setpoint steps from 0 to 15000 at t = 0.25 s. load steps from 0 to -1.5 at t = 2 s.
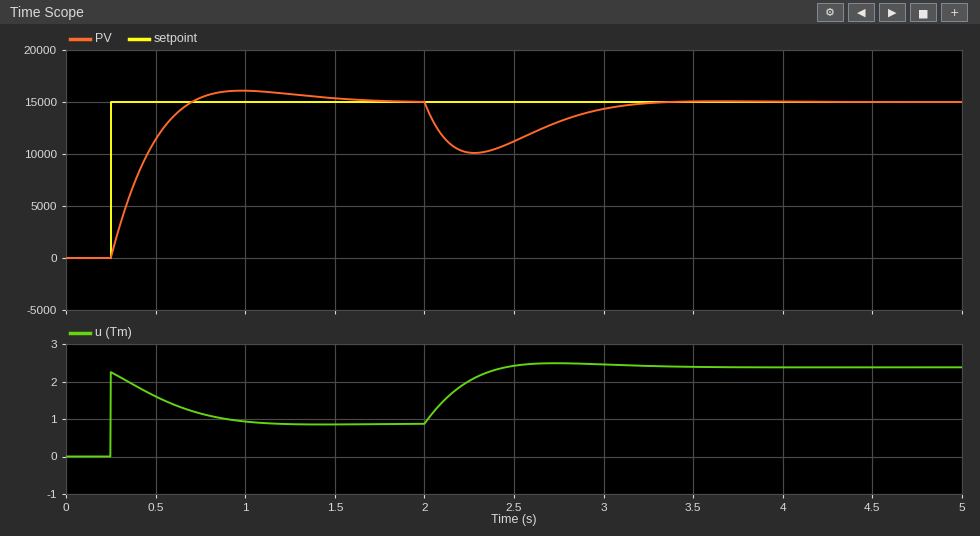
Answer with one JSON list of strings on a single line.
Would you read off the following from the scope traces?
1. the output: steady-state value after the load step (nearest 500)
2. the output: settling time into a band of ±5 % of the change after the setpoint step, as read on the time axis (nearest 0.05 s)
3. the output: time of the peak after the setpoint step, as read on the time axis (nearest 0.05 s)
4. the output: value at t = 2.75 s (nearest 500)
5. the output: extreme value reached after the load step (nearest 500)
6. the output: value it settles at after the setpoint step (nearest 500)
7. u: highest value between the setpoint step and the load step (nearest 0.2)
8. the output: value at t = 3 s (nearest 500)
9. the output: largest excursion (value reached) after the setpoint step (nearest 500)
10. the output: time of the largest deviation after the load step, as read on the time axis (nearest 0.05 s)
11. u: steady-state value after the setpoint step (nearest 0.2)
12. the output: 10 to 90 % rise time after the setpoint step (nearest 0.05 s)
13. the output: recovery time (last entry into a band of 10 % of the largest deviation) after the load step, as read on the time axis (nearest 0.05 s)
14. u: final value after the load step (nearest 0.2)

["15000", "1.25 s", "1.00 s", "13000", "10000", "15000", "2.2", "14500", "16000", "2.30 s", "0.8", "0.30 s", "3.05 s", "2.4"]
